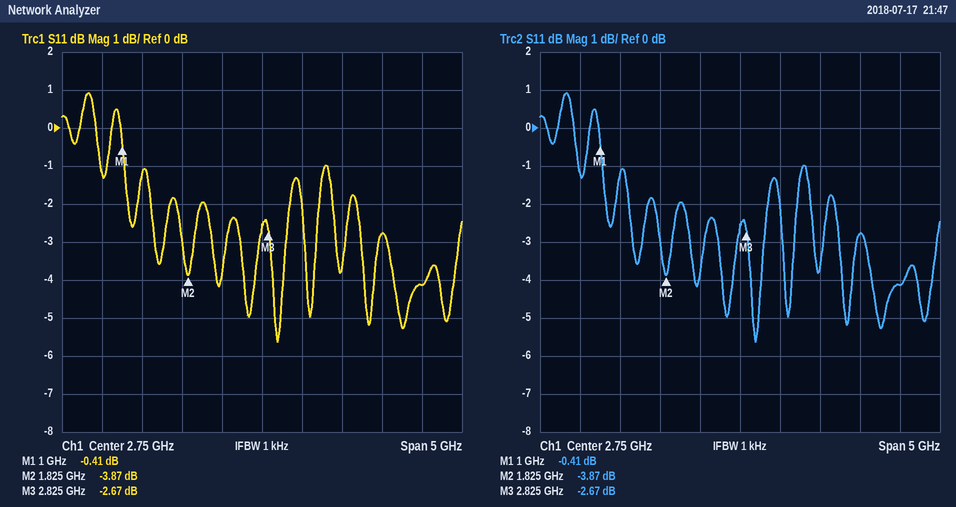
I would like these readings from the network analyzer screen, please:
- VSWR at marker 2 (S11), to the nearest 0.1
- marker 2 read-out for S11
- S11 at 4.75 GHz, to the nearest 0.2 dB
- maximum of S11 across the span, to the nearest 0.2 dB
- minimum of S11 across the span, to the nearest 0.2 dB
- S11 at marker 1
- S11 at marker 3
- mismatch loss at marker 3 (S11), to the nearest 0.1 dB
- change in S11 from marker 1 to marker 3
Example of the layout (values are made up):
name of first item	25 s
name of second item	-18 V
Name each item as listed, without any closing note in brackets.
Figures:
VSWR at marker 2 (S11), to the nearest 0.1	4.6
marker 2 read-out for S11	-3.87 dB
S11 at 4.75 GHz, to the nearest 0.2 dB	-4.2 dB
maximum of S11 across the span, to the nearest 0.2 dB	1.0 dB
minimum of S11 across the span, to the nearest 0.2 dB	-5.6 dB
S11 at marker 1	-0.41 dB
S11 at marker 3	-2.67 dB
mismatch loss at marker 3 (S11), to the nearest 0.1 dB	3.4 dB
change in S11 from marker 1 to marker 3	-2.26 dB
